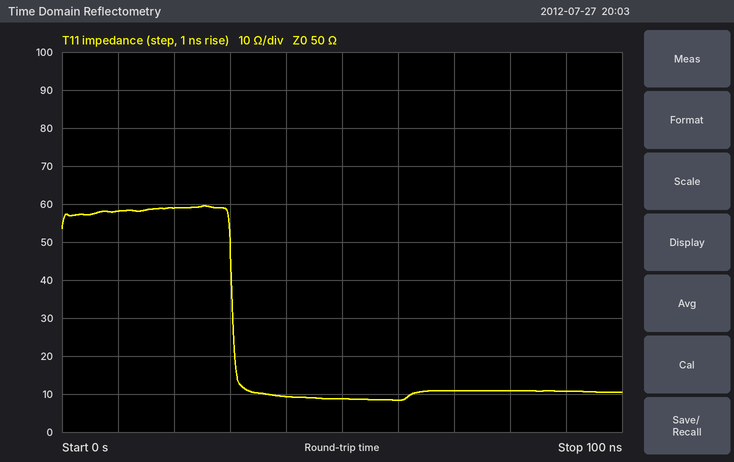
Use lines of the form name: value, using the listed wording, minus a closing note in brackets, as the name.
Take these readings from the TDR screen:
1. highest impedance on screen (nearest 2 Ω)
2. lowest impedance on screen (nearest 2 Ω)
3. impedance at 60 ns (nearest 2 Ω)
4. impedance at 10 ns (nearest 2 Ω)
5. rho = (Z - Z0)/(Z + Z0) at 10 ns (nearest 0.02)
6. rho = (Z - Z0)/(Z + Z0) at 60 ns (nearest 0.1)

highest impedance on screen: 60 Ω
lowest impedance on screen: 8 Ω
impedance at 60 ns: 8 Ω
impedance at 10 ns: 58 Ω
rho = (Z - Z0)/(Z + Z0) at 10 ns: +0.08
rho = (Z - Z0)/(Z + Z0) at 60 ns: -0.7
